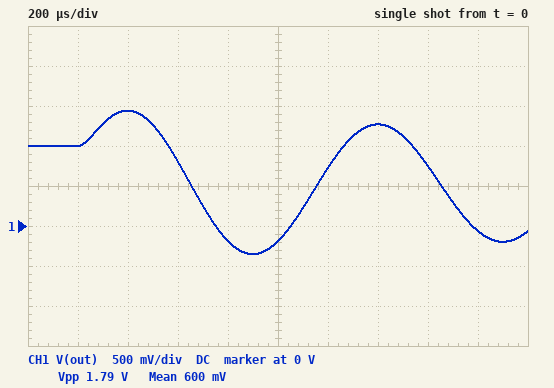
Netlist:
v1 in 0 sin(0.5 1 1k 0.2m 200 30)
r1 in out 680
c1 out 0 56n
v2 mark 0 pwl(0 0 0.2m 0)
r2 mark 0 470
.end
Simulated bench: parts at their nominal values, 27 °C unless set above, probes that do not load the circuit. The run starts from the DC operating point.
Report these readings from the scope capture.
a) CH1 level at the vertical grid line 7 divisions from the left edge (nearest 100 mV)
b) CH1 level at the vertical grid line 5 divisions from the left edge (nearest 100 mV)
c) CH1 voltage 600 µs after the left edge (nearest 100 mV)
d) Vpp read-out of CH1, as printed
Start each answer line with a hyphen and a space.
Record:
- 1.3 V
- -200 mV
- 800 mV
- 1.79 V
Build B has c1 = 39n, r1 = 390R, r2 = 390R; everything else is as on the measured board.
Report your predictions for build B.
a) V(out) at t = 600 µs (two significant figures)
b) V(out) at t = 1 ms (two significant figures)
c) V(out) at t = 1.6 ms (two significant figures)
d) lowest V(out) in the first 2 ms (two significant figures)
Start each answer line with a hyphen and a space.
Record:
- 680 mV
- -130 mV
- 650 mV
- -370 mV
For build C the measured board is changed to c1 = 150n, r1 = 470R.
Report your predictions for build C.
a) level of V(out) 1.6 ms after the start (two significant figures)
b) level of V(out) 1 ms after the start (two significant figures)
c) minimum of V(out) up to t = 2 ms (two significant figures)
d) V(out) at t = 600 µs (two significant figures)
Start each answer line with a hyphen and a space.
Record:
- 850 mV
- -220 mV
- -300 mV
- 930 mV
